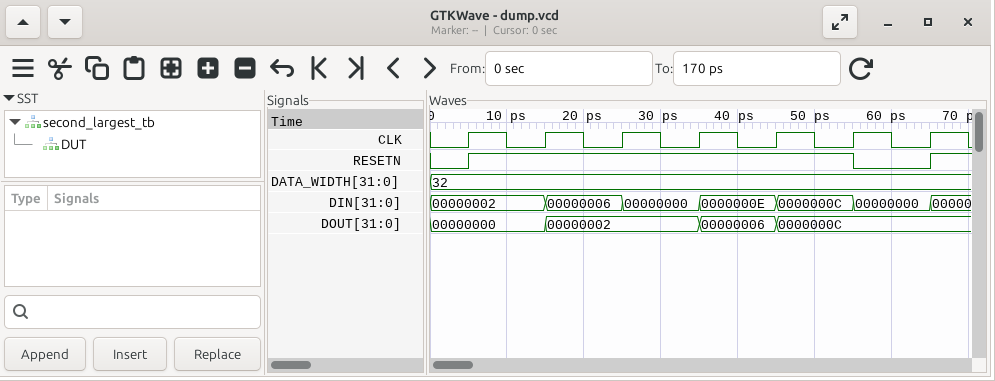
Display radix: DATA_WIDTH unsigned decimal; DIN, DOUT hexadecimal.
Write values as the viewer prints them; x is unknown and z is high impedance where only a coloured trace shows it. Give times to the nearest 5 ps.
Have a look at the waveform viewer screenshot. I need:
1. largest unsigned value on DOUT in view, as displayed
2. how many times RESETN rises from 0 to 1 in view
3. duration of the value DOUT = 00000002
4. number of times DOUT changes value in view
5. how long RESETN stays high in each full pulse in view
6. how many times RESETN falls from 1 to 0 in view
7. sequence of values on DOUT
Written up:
0000000C
2
20 ps
3
50 ps
1
00000000, 00000002, 00000006, 0000000C
